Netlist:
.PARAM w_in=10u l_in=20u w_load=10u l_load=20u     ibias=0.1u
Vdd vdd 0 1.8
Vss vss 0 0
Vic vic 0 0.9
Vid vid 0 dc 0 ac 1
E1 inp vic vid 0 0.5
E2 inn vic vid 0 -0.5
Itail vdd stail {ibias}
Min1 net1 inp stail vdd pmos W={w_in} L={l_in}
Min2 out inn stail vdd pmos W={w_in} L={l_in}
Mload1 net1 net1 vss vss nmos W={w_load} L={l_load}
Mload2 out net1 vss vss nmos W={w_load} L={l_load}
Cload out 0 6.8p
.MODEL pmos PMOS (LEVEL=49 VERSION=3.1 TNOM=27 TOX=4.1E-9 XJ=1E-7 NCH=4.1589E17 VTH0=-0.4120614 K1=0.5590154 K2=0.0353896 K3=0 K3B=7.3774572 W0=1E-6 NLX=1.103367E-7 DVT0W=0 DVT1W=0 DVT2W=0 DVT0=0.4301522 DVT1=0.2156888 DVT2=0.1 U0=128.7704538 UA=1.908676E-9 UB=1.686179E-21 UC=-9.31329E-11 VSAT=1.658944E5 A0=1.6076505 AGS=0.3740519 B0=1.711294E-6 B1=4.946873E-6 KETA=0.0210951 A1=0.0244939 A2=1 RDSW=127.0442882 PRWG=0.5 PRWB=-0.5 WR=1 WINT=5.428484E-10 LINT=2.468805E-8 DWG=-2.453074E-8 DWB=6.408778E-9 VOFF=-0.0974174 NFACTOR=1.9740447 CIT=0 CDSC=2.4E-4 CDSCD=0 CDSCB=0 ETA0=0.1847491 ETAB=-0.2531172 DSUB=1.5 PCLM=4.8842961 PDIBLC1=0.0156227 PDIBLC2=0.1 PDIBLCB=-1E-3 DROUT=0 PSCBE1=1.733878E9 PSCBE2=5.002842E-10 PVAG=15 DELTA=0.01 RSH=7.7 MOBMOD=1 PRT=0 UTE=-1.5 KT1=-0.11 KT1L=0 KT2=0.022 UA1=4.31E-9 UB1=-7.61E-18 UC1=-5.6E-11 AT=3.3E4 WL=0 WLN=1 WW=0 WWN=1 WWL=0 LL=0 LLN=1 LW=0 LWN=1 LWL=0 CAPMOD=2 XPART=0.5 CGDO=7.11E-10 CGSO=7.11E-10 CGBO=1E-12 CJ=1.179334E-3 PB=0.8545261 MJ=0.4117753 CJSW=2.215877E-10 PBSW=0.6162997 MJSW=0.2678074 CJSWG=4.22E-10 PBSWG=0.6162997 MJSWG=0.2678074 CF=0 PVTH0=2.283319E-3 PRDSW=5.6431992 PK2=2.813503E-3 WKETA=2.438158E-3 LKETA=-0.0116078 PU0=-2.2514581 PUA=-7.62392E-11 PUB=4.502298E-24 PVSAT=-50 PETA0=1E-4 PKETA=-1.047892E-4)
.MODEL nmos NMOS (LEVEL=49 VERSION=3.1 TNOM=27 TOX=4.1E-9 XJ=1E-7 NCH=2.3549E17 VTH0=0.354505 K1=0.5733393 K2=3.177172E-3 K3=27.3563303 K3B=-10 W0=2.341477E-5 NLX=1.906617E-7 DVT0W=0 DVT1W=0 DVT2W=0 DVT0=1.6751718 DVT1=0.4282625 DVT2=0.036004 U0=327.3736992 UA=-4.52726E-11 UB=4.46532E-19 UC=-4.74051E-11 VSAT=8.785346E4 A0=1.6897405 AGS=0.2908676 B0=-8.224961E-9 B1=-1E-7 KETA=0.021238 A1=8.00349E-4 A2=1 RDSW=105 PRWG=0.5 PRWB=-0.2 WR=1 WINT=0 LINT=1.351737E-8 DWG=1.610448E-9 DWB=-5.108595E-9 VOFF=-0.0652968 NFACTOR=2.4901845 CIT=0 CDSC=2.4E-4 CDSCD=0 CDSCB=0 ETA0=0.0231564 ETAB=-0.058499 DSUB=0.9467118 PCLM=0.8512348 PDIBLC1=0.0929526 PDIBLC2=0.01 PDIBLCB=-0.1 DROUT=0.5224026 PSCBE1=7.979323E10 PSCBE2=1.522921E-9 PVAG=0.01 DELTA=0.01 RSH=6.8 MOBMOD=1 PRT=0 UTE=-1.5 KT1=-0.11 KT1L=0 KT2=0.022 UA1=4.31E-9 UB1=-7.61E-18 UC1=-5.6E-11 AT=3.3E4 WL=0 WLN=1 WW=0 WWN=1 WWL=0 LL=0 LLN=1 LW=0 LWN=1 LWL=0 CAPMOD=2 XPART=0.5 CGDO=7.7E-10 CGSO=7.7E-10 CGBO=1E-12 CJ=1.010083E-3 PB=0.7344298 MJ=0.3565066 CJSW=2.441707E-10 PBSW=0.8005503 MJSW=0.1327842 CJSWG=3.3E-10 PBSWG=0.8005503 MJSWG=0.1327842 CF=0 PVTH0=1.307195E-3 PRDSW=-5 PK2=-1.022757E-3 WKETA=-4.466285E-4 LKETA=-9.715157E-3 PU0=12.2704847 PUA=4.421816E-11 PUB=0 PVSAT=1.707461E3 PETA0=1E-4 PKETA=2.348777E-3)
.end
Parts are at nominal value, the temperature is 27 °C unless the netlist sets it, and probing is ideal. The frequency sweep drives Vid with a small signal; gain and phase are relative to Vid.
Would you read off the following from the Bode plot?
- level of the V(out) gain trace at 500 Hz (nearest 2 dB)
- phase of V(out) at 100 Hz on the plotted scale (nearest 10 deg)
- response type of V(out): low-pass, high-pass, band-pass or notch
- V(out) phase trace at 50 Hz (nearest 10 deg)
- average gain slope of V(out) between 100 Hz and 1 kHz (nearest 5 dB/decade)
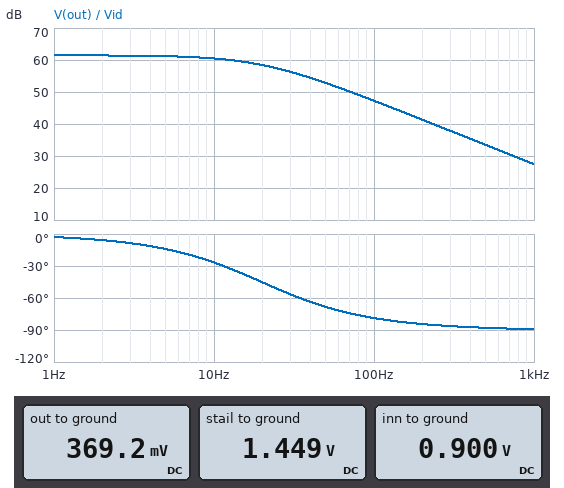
34 dB
-80 deg
low-pass
-70 deg
-20 dB/decade
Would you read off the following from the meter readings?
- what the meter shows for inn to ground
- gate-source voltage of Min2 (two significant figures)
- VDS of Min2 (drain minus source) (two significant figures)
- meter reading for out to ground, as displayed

0.900 V
-550 mV
-1.1 V
369.2 mV
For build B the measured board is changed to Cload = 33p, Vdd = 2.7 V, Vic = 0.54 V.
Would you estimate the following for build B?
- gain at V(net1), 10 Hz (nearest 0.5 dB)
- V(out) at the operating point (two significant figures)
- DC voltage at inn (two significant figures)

-7.5 dB
370 mV
540 mV
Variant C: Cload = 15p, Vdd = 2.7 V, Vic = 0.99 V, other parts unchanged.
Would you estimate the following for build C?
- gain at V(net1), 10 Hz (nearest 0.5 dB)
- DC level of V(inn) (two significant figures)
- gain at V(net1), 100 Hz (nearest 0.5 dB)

-7.5 dB
990 mV
-7.5 dB
